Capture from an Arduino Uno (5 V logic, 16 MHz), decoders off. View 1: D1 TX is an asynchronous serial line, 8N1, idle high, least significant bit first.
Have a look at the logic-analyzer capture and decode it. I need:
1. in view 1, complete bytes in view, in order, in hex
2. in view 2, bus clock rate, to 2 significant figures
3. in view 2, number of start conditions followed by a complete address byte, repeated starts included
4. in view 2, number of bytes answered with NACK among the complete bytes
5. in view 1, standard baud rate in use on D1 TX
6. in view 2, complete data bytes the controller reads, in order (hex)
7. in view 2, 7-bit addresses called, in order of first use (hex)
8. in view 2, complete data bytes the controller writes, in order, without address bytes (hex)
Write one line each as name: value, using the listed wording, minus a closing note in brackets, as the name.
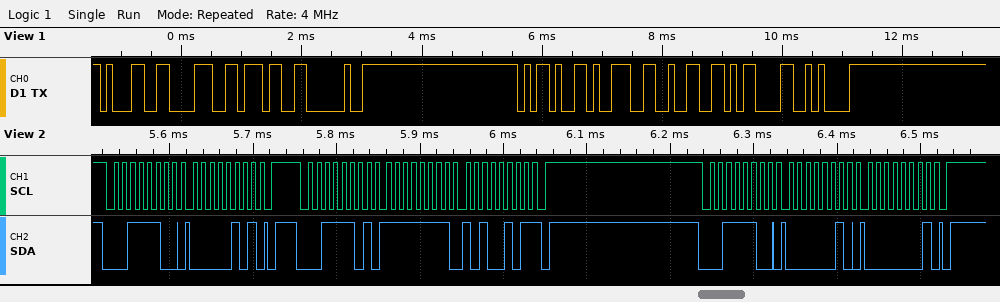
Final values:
in view 1, complete bytes in view, in order, in hex: 31 38 37 20 2D 39 32 0D 0A
in view 2, bus clock rate, to 2 significant figures: 100 kHz
in view 2, number of start conditions followed by a complete address byte, repeated starts included: 3
in view 2, number of bytes answered with NACK among the complete bytes: 1
in view 1, standard baud rate in use on D1 TX: 9600 baud
in view 2, complete data bytes the controller reads, in order: FF A5
in view 2, 7-bit addresses called, in order of first use: 0x1E
in view 2, complete data bytes the controller writes, in order, without address bytes: 05 02 01
